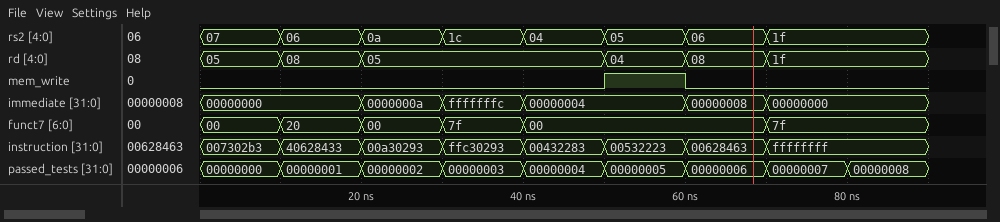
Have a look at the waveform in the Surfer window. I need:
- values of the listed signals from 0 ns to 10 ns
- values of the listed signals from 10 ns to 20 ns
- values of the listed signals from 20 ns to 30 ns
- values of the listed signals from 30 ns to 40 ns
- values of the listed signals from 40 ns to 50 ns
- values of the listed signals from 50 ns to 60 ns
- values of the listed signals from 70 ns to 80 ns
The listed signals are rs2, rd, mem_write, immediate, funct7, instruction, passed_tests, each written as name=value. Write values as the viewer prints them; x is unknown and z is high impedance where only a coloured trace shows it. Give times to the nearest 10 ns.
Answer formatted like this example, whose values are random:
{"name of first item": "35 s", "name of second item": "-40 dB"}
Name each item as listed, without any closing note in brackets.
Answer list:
{"values of the listed signals from 0 ns to 10 ns": "rs2=07, rd=05, mem_write=0, immediate=00000000, funct7=00, instruction=007302b3, passed_tests=00000000", "values of the listed signals from 10 ns to 20 ns": "rs2=06, rd=08, mem_write=0, immediate=00000000, funct7=20, instruction=40628433, passed_tests=00000001", "values of the listed signals from 20 ns to 30 ns": "rs2=0a, rd=05, mem_write=0, immediate=0000000a, funct7=00, instruction=00a30293, passed_tests=00000002", "values of the listed signals from 30 ns to 40 ns": "rs2=1c, rd=05, mem_write=0, immediate=fffffffc, funct7=7f, instruction=ffc30293, passed_tests=00000003", "values of the listed signals from 40 ns to 50 ns": "rs2=04, rd=05, mem_write=0, immediate=00000004, funct7=00, instruction=00432283, passed_tests=00000004", "values of the listed signals from 50 ns to 60 ns": "rs2=05, rd=04, mem_write=1, immediate=00000004, funct7=00, instruction=00532223, passed_tests=00000005", "values of the listed signals from 70 ns to 80 ns": "rs2=1f, rd=1f, mem_write=0, immediate=00000000, funct7=7f, instruction=ffffffff, passed_tests=00000007"}
